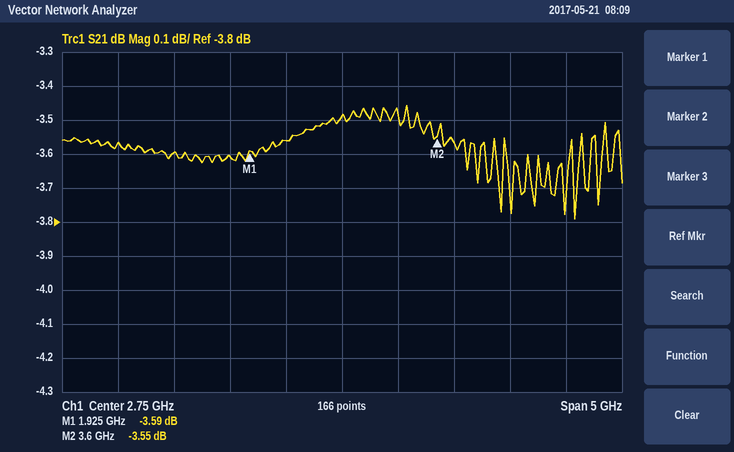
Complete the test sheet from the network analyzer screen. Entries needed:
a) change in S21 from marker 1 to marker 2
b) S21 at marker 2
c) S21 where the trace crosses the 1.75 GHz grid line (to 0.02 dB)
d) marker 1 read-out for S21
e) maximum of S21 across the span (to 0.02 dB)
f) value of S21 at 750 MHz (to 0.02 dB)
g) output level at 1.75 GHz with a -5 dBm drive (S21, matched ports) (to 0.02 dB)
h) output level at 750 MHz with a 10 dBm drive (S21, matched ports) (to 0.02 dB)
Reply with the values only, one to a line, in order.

0.04 dB
-3.55 dB
-3.60 dB
-3.59 dB
-3.46 dB
-3.56 dB
-8.60 dBm
6.44 dBm
